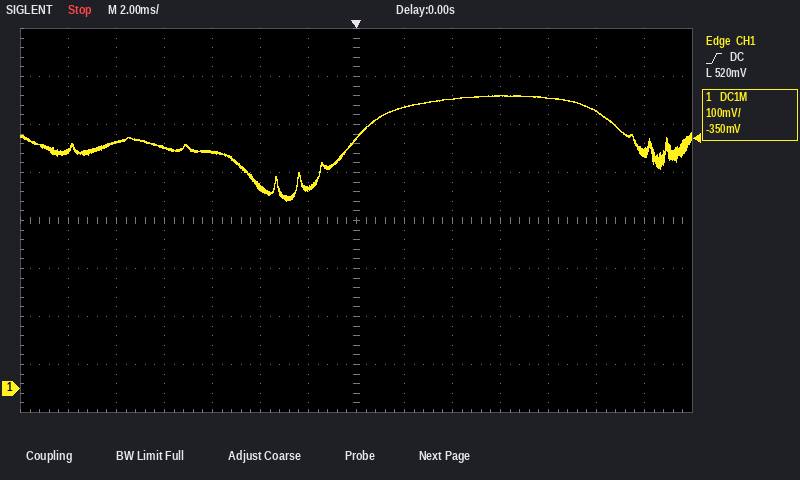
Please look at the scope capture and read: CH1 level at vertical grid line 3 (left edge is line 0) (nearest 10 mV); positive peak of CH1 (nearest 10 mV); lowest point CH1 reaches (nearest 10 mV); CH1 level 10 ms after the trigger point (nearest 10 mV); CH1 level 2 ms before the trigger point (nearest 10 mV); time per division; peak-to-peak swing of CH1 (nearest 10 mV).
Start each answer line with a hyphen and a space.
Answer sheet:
- 500 mV
- 610 mV
- 390 mV
- 580 mV
- 420 mV
- 2 ms
- 220 mV
